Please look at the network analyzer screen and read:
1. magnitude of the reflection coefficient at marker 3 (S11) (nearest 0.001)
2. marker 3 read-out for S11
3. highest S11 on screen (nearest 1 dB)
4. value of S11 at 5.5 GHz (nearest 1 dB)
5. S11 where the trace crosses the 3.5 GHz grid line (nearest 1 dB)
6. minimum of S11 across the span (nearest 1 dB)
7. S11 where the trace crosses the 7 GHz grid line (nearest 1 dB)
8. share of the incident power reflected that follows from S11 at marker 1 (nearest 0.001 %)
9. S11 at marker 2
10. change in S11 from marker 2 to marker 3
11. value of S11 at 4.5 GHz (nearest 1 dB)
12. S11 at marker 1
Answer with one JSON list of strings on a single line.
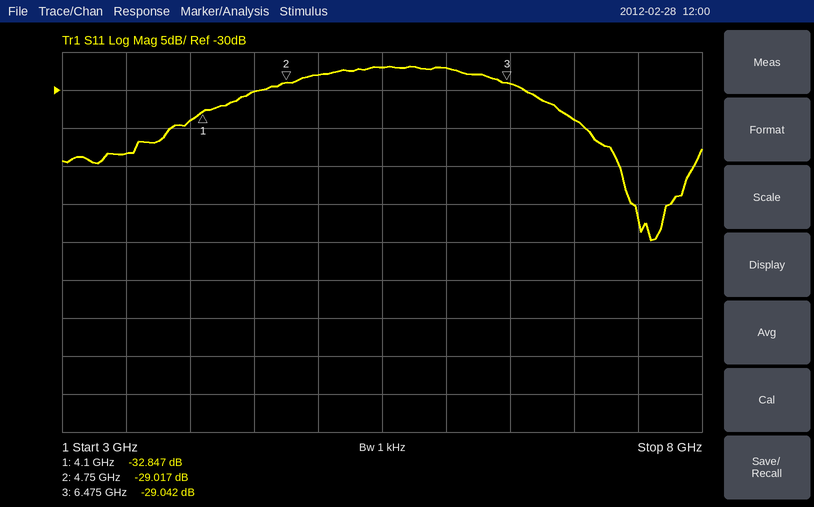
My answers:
["0.035", "-29.042 dB", "-27 dB", "-27 dB", "-38 dB", "-50 dB", "-34 dB", "0.052 %", "-29.017 dB", "-0.025 dB", "-30 dB", "-32.847 dB"]
